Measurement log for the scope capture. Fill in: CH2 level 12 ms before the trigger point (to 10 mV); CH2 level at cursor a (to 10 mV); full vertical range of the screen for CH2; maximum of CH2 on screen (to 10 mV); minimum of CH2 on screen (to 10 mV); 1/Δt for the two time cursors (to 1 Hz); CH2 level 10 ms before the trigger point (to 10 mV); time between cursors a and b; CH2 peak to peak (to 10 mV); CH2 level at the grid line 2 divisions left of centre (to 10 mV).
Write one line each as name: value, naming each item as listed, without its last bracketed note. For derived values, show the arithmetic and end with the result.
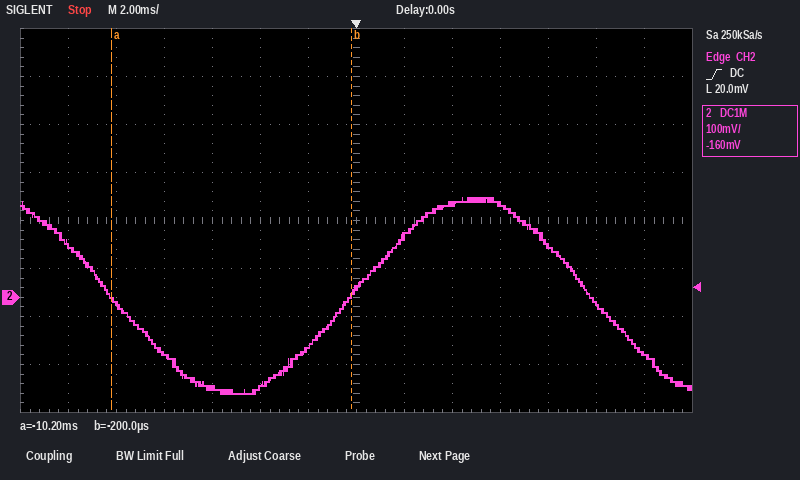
CH2 level 12 ms before the trigger point: 110 mV
CH2 level at cursor a: 0 mV
full vertical range of the screen for CH2: 800 mV
maximum of CH2 on screen: 210 mV
minimum of CH2 on screen: -200 mV
1/Δt for the two time cursors: 1 / 10.0 ms ≈ 100 Hz
CH2 level 10 ms before the trigger point: -20 mV
time between cursors a and b: -200 µs − (-10.2 ms) = 10.0 ms
CH2 peak to peak: 210 mV − (-200 mV) = 410 mV
CH2 level at the grid line 2 divisions left of centre: -190 mV
